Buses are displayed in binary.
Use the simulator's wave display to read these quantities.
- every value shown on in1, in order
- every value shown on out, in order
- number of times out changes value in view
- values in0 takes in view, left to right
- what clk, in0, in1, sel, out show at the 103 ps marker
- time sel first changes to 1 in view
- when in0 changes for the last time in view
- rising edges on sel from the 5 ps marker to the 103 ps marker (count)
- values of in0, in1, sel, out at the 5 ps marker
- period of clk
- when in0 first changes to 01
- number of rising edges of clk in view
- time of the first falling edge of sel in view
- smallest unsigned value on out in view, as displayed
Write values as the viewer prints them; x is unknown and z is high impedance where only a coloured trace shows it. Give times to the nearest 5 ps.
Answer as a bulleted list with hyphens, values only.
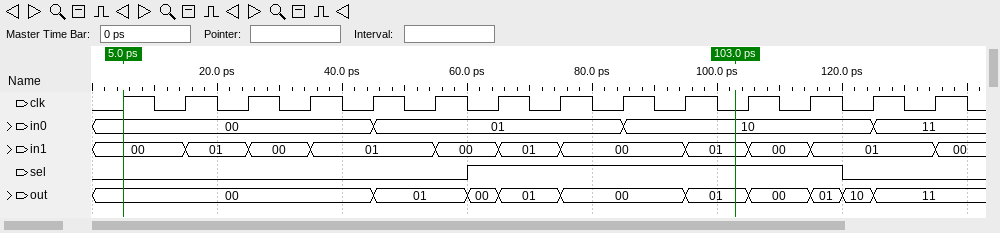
- 00, 01, 00, 01, 00, 01, 00, 01, 00, 01, 00
- 00, 01, 00, 01, 00, 01, 00, 01, 10, 11
- 9
- 00, 01, 10, 11
- clk=0, in0=10, in1=01, sel=1, out=01
- 60 ps
- 125 ps
- 1
- in0=00, in1=00, sel=0, out=00
- 10 ps
- 45 ps
- 14
- 120 ps
- 00
